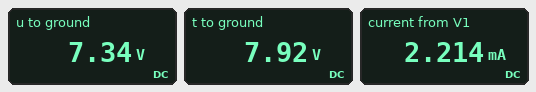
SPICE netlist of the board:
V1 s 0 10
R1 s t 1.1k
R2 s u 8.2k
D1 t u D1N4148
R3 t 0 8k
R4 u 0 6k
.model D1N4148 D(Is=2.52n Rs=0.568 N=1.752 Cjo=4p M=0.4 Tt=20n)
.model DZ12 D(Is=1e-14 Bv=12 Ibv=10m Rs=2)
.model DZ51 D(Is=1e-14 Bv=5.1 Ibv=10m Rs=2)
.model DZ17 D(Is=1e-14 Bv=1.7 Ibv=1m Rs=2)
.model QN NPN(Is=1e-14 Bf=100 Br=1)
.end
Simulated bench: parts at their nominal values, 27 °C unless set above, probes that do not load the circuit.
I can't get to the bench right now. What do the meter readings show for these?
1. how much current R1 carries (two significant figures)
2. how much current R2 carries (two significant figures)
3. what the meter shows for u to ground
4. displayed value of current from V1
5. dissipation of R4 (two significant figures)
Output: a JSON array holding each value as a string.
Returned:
["1.9 mA", "320 µA", "7.34 V", "2.214 mA", "9.0 mW"]
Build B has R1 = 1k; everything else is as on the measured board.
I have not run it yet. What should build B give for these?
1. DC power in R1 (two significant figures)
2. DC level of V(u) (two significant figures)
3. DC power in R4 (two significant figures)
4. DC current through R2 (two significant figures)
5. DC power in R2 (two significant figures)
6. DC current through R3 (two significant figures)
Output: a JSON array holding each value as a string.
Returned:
["3.8 mW", "7.5 V", "9.3 mW", "310 µA", "780 µW", "1.0 mA"]
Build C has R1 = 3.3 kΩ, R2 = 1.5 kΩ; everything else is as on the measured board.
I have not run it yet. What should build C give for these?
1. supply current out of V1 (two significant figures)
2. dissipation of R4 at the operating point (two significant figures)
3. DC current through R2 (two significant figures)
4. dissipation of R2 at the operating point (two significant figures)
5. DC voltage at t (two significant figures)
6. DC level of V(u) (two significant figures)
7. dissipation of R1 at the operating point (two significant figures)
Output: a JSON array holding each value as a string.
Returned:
["2.2 mA", "11 mW", "1.3 mA", "2.7 mW", "7.1 V", "8.0 V", "2.6 mW"]
